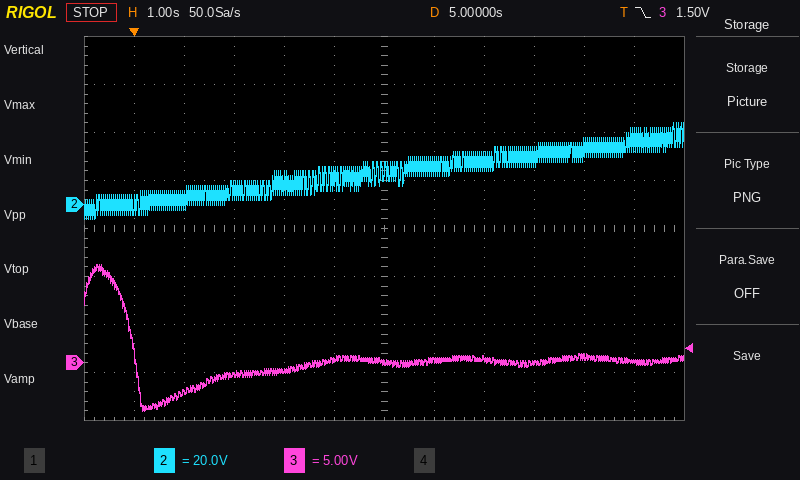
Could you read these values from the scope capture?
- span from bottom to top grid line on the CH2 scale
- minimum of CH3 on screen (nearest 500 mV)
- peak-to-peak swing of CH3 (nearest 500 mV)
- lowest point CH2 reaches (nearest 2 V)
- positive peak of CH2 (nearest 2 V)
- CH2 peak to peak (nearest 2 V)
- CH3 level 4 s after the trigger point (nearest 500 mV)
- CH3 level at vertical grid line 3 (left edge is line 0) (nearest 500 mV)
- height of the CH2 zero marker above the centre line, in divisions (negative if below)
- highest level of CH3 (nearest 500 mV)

160 V
-5.0 V
15.0 V
-6 V
34 V
40 V
500 mV
-1.0 V
+0.5 div
10.0 V
